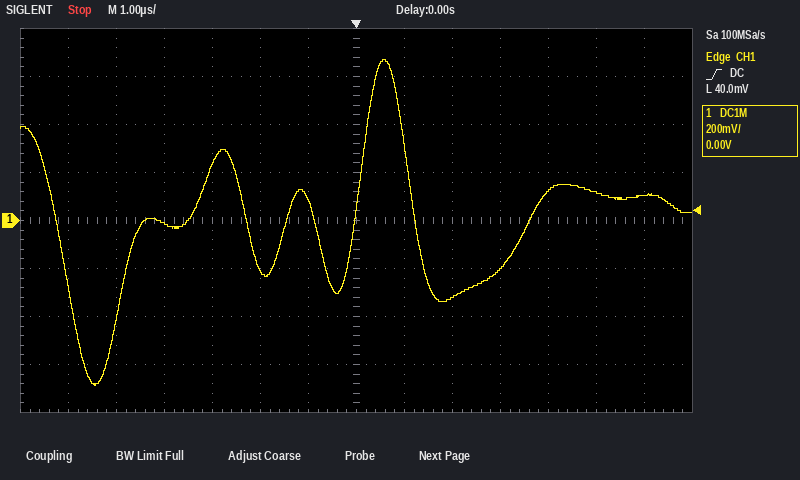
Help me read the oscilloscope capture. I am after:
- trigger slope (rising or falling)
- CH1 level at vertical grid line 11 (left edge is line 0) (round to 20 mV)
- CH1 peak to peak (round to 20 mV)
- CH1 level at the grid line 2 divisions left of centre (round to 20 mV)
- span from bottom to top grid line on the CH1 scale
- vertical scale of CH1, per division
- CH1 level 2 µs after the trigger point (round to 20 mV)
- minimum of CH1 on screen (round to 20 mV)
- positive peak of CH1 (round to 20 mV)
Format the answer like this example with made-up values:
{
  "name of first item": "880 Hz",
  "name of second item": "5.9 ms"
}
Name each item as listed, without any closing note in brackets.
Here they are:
{
  "trigger slope": "rising",
  "CH1 level at vertical grid line 11 (left edge is line 0)": "120 mV",
  "CH1 peak to peak": "1.36 V",
  "CH1 level at the grid line 2 divisions left of centre": "-200 mV",
  "span from bottom to top grid line on the CH1 scale": "1.6 V",
  "vertical scale of CH1, per division": "200 mV",
  "CH1 level 2 µs after the trigger point": "-320 mV",
  "minimum of CH1 on screen": "-680 mV",
  "positive peak of CH1": "680 mV"
}
